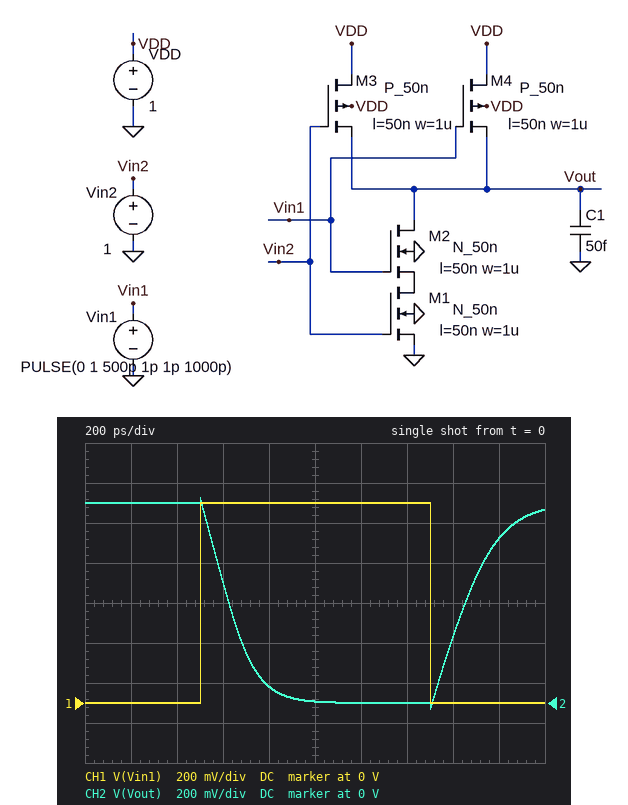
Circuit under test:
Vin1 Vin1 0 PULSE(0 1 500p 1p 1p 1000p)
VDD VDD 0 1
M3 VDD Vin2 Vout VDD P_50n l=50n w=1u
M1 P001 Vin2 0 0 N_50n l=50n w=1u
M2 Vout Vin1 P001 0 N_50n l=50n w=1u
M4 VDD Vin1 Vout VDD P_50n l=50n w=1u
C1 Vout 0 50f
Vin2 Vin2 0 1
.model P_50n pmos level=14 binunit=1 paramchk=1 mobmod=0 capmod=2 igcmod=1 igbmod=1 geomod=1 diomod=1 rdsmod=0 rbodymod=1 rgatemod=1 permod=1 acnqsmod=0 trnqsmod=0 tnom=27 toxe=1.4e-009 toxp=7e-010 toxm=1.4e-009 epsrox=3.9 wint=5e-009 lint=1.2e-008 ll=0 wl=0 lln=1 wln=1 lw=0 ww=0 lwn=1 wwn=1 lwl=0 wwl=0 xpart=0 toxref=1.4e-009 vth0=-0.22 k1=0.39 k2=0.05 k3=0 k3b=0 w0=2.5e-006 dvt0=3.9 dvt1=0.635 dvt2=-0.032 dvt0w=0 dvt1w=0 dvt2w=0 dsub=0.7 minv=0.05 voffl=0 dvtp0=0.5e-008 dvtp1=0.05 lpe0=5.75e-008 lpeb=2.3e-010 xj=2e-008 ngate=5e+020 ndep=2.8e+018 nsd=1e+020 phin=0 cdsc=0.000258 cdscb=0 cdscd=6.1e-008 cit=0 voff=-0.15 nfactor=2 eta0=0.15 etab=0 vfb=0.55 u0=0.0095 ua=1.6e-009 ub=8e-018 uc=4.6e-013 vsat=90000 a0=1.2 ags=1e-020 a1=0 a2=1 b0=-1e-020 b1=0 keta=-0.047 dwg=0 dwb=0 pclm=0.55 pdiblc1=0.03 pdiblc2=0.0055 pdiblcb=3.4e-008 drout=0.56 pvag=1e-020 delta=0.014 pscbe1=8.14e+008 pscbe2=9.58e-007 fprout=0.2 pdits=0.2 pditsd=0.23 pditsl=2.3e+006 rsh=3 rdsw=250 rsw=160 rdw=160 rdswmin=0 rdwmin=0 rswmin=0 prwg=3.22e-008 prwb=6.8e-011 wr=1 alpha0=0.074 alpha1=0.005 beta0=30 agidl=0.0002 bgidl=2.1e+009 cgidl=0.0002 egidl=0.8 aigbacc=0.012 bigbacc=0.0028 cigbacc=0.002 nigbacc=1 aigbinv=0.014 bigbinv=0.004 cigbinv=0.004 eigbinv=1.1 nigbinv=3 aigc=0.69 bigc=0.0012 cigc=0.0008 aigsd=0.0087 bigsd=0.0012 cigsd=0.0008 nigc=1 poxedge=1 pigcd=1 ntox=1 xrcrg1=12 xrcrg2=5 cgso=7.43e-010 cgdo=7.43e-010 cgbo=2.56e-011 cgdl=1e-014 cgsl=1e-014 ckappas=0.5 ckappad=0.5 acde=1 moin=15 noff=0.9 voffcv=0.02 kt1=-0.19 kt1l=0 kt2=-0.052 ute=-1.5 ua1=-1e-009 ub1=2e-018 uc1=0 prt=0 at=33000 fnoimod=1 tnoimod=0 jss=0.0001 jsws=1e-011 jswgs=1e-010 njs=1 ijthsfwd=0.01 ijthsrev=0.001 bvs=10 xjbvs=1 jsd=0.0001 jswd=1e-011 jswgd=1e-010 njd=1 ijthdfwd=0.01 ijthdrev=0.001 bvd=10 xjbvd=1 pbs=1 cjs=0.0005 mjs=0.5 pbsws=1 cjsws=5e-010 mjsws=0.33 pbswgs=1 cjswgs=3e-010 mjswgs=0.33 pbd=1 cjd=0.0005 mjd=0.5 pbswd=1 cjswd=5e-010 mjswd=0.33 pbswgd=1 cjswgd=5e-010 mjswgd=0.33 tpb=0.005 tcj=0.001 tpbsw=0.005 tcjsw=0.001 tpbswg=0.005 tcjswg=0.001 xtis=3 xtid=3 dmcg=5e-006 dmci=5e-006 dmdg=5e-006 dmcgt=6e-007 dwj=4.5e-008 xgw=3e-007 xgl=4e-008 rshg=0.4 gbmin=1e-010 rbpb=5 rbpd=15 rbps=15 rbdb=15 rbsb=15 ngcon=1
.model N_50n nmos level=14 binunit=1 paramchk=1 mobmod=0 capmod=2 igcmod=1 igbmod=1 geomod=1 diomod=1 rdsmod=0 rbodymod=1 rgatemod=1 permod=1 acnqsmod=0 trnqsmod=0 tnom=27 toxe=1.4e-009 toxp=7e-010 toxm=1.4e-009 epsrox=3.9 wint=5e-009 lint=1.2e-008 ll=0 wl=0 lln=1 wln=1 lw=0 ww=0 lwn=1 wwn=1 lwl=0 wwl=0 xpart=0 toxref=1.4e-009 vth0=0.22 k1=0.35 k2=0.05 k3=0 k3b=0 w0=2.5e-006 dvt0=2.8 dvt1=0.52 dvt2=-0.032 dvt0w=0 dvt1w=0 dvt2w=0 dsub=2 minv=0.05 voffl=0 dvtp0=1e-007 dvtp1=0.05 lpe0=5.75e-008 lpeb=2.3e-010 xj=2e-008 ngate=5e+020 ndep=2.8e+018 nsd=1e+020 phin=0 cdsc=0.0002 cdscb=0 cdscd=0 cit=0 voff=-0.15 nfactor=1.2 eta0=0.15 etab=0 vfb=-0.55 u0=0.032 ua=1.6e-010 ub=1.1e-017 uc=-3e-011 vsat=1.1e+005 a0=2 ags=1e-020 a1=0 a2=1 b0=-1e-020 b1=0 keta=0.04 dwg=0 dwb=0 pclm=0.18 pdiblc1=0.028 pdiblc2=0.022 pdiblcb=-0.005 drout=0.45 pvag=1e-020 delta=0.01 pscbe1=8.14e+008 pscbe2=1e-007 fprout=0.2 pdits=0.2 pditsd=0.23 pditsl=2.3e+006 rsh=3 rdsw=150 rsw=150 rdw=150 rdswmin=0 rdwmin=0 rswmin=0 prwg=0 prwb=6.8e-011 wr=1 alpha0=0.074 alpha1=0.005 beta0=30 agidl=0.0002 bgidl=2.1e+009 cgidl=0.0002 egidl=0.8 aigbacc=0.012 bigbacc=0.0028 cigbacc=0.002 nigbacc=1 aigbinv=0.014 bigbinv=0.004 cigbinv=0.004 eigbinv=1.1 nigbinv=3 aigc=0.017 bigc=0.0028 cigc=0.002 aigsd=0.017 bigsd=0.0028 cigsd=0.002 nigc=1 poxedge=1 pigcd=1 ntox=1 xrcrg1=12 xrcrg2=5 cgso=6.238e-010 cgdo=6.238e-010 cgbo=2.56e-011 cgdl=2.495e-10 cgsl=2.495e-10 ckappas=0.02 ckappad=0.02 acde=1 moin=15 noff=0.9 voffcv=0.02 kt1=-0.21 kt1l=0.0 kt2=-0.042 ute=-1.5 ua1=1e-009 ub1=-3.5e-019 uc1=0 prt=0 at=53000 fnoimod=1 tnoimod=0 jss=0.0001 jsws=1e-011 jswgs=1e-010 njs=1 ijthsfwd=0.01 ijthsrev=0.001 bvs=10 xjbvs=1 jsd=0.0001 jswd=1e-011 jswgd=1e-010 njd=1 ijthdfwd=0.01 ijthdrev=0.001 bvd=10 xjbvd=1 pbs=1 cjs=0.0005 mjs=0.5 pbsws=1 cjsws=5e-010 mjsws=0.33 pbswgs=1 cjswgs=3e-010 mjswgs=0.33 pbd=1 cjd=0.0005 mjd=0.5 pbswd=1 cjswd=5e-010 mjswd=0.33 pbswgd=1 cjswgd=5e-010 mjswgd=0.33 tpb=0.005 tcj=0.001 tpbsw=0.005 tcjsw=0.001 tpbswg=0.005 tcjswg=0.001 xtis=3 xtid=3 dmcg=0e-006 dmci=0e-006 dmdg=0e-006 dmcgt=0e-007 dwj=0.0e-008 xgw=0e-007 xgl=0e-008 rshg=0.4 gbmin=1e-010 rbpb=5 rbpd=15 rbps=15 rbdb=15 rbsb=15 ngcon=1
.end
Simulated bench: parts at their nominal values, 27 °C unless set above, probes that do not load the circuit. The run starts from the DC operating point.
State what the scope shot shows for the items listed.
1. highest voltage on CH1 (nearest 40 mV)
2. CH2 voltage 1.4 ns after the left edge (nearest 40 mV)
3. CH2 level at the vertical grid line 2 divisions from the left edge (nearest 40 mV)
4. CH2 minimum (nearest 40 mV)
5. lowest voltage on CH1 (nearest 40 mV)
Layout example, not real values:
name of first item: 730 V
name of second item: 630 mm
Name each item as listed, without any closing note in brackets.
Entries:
highest voltage on CH1: 1.00 V
CH2 voltage 1.4 ns after the left edge: 0 V
CH2 level at the vertical grid line 2 divisions from the left edge: 1.00 V
CH2 minimum: -40 mV
lowest voltage on CH1: 0 V
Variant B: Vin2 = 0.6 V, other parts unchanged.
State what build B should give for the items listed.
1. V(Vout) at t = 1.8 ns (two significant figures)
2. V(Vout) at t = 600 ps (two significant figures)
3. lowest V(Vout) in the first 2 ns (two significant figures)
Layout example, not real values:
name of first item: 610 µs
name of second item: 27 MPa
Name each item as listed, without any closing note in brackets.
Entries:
V(Vout) at t = 1.8 ns: 860 mV
V(Vout) at t = 600 ps: 800 mV
lowest V(Vout) in the first 2 ns: 4.1 mV
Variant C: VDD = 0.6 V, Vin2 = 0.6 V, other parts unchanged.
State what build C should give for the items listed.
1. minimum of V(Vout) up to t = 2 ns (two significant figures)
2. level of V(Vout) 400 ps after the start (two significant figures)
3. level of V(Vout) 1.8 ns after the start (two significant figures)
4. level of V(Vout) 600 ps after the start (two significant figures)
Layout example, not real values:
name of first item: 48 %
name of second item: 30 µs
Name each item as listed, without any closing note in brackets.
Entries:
minimum of V(Vout) up to t = 2 ns: -29 mV
level of V(Vout) 400 ps after the start: 600 mV
level of V(Vout) 1.8 ns after the start: 280 mV
level of V(Vout) 600 ps after the start: 410 mV
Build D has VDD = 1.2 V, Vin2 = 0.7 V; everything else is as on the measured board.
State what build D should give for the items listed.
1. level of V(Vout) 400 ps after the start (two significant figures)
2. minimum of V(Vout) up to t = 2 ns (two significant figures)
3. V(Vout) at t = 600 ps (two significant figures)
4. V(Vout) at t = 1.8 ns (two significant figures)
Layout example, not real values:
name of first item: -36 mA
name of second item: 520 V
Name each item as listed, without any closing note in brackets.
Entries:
level of V(Vout) 400 ps after the start: 1.2 V
minimum of V(Vout) up to t = 2 ns: 58 mV
V(Vout) at t = 600 ps: 930 mV
V(Vout) at t = 1.8 ns: 1.1 V
